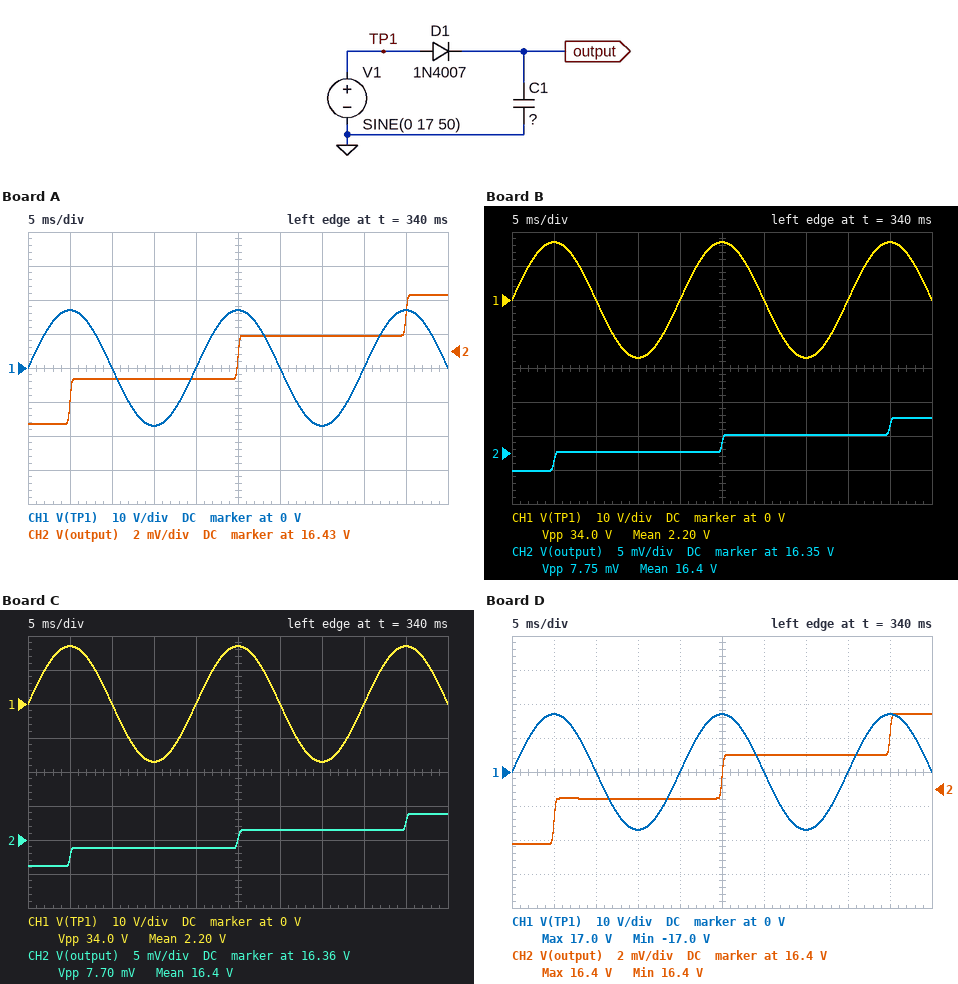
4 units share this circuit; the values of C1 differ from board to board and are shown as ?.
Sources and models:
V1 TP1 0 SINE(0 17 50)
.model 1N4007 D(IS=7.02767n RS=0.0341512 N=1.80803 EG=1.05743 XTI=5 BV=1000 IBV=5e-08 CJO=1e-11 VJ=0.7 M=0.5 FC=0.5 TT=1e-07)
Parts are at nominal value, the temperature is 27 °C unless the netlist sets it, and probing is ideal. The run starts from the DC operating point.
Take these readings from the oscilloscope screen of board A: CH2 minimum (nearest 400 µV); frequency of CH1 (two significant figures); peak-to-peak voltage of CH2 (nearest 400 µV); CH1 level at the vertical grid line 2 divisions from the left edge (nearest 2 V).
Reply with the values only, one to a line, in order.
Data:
16.4276 V
50 Hz
7.6 mV
0 V
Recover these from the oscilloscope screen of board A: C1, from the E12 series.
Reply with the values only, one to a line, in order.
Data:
220 µF
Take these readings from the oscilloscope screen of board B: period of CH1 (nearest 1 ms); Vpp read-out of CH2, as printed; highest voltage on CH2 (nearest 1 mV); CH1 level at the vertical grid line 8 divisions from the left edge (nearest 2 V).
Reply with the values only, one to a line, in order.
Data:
20 ms
7.75 mV
16.355 V
0 V
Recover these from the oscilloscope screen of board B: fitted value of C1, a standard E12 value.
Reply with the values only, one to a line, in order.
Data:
1.2 mF
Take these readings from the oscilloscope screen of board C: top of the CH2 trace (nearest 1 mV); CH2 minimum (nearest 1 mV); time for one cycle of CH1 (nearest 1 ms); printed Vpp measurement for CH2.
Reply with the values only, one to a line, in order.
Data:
16.364 V
16.356 V
20 ms
7.70 mV
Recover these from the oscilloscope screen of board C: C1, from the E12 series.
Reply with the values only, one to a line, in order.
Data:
1 mF
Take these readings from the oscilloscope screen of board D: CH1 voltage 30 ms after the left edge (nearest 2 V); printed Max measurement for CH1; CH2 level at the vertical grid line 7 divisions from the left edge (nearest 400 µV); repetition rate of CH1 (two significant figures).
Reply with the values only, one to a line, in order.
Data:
0 V
17.0 V
16.4060 V
50 Hz
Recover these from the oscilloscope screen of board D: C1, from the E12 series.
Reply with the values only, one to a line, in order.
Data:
390 µF
